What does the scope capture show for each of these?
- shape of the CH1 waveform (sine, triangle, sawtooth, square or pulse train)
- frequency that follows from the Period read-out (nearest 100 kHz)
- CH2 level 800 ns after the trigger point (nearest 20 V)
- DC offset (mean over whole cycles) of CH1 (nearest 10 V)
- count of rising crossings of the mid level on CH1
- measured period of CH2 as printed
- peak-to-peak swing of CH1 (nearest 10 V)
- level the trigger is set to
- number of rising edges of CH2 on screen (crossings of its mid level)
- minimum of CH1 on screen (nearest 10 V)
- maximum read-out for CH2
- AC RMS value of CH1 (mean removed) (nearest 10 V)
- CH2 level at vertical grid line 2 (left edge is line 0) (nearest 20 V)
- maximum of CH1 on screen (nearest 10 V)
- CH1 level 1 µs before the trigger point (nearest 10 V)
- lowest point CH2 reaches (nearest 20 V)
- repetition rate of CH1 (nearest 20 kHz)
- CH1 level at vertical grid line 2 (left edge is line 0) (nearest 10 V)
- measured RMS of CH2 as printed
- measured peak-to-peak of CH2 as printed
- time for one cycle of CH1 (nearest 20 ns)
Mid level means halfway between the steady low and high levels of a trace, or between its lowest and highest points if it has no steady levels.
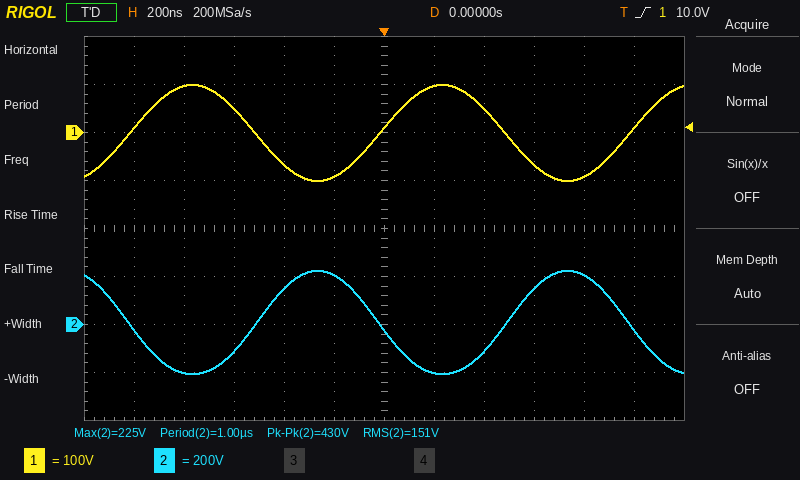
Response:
sine
1.0 MHz
200 V
0 V
3
1.00 µs
200 V
10.0 V
2
-100 V
225 V
70 V
-200 V
100 V
10 V
-200 V
1.00 MHz
100 V
151 V
430 V
1.00 µs
